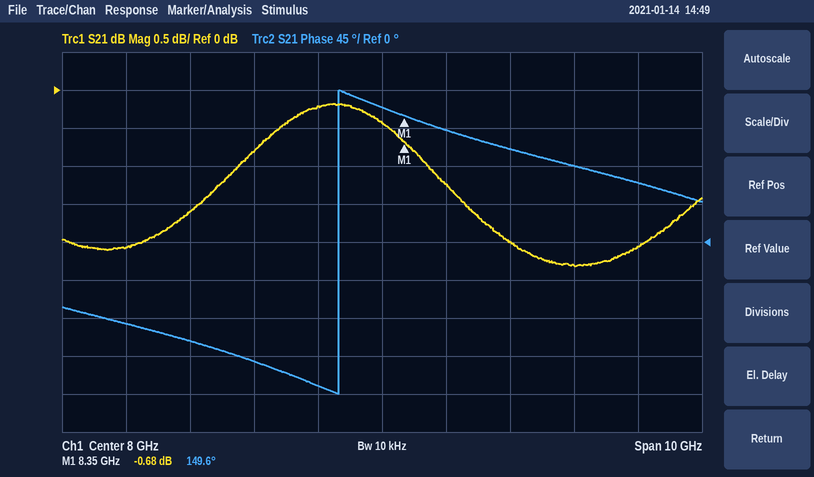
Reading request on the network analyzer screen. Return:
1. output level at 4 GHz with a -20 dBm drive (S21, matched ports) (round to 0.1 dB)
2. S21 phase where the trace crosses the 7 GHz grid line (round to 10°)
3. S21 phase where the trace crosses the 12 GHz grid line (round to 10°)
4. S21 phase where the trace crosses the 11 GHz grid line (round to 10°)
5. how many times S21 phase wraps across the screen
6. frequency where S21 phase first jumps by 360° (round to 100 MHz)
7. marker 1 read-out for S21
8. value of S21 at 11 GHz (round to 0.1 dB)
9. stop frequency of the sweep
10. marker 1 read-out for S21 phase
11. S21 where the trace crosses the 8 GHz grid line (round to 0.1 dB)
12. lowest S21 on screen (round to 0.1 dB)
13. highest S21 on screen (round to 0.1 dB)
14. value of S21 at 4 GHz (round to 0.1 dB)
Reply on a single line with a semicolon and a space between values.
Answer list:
-22.1 dBm; -170°; 70°; 90°; 1; 7.3 GHz; -0.68 dB; -2.3 dB; 13 GHz; 149.6°; -0.4 dB; -2.3 dB; -0.2 dB; -2.1 dB
